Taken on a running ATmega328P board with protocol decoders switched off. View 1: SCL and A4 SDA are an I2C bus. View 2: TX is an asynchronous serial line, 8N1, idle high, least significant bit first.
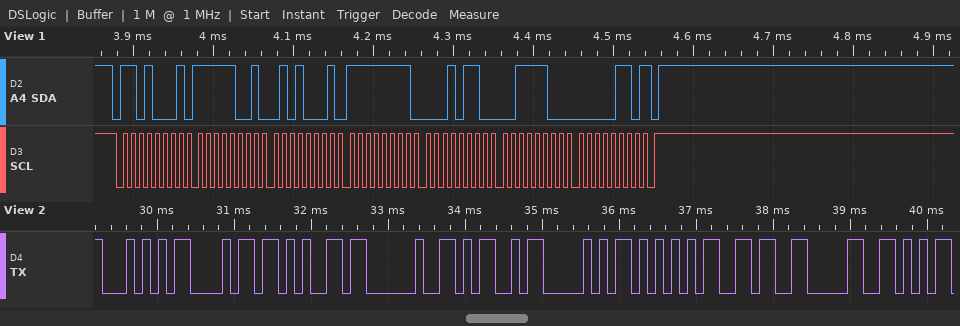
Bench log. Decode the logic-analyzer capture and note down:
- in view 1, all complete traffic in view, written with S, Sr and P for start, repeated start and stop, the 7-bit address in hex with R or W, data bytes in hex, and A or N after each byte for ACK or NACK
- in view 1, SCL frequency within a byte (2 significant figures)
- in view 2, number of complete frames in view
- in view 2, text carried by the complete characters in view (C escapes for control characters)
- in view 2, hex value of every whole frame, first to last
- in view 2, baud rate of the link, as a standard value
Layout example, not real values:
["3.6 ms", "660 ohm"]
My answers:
["S 68R A F9 A 51 A FF A 16 A 3C A 06 N P", "100 kHz", "9", "\"The MPU60\"", "0x54 0x68 0x65 0x20 0x4D 0x50 0x55 0x36 0x30", "9600 baud"]
